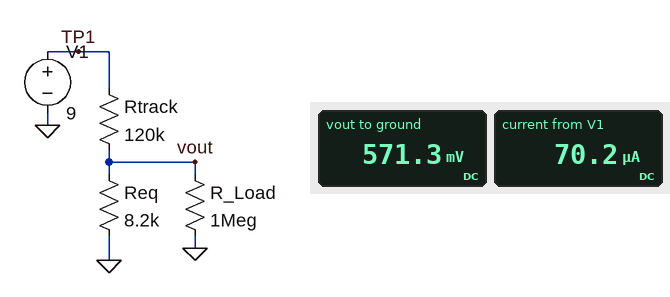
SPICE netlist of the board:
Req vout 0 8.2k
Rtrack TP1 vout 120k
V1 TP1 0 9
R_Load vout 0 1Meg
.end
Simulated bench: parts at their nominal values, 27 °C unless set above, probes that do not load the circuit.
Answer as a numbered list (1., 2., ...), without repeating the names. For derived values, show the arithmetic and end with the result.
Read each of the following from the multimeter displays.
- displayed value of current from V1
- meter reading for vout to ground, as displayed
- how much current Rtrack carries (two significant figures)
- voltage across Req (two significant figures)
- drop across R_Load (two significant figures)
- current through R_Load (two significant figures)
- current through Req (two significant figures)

1. 70.2 µA
2. 571.3 mV
3. (9 V - 571.3 mV) / 120 kΩ = 70 µA
4. 571.3 mV = 570 mV
5. 571.3 mV = 570 mV
6. (571.3 mV) / 1 MΩ = 570 nA
7. (571.3 mV) / 8.2 kΩ = 70 µA
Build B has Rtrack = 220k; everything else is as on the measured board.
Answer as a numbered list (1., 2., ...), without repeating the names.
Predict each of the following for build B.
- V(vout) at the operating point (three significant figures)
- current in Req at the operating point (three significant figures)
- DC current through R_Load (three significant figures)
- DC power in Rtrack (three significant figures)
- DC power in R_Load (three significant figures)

1. 321 mV
2. 39.1 µA
3. 321 nA
4. 342 µW
5. 103 nW
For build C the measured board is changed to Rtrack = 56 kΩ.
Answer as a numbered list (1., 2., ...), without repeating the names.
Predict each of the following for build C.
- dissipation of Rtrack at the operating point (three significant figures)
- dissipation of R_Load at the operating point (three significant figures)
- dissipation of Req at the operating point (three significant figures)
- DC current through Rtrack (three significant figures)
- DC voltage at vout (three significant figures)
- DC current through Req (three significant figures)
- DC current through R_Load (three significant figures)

1. 1.10 mW
2. 1.30 µW
3. 159 µW
4. 140 µA
5. 1.14 V
6. 139 µA
7. 1.14 µA
